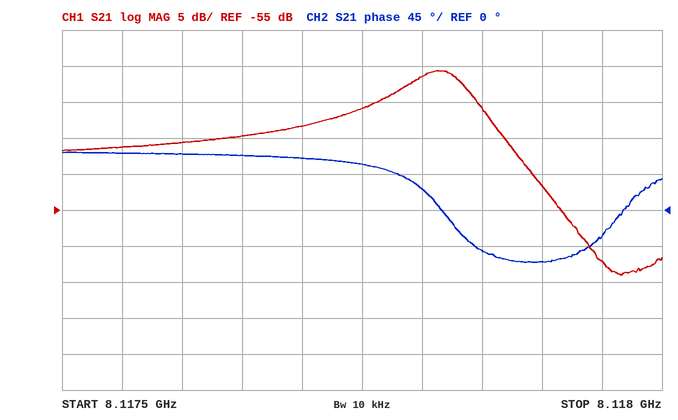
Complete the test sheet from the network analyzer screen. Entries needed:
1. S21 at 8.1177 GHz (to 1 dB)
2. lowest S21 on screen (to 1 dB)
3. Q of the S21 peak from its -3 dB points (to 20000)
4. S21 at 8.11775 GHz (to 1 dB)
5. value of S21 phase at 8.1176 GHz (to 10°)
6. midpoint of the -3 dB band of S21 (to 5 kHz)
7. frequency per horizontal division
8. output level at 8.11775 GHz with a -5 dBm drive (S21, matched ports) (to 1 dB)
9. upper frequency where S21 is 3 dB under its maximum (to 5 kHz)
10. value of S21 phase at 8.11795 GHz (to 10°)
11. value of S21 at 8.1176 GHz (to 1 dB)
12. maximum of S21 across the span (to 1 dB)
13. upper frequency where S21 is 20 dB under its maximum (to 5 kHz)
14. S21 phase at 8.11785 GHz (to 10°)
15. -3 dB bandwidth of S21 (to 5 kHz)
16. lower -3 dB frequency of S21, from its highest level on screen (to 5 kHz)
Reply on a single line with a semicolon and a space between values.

-43 dB; -64 dB; 140000; -41 dB; 70°; 8.117810 GHz; 50 kHz; -46 dBm; 8.117840 GHz; -30°; -46 dB; -36 dB; 8.117920 GHz; -50°; 60 kHz; 8.117780 GHz
